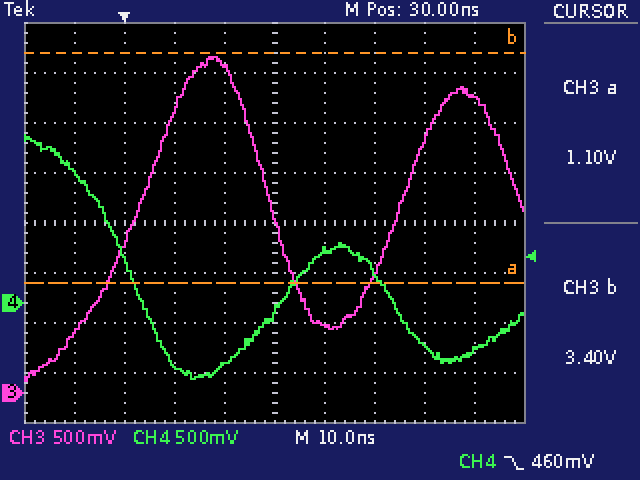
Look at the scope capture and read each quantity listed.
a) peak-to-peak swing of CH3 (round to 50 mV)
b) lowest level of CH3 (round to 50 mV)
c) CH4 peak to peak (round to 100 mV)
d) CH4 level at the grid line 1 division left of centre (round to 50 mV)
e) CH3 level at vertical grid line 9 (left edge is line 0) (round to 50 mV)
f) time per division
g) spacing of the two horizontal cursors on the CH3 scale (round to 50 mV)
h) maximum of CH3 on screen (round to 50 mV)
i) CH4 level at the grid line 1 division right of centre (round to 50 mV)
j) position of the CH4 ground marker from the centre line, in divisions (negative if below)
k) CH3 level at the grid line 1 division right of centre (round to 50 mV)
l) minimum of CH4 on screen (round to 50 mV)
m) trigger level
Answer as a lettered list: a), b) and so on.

a) 3.25 V
b) 100 mV
c) 2.40 V
d) -600 mV
e) 2.95 V
f) 10 ns
g) 2.30 V
h) 3.35 V
i) 500 mV
j) -1.6 div
k) 700 mV
l) -750 mV
m) 460 mV
